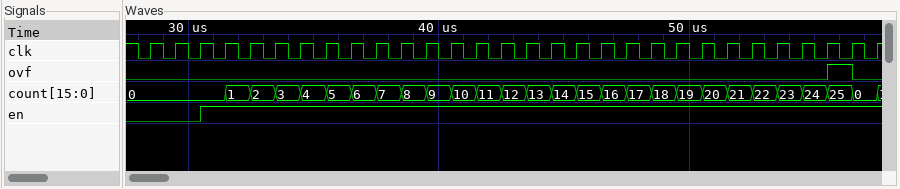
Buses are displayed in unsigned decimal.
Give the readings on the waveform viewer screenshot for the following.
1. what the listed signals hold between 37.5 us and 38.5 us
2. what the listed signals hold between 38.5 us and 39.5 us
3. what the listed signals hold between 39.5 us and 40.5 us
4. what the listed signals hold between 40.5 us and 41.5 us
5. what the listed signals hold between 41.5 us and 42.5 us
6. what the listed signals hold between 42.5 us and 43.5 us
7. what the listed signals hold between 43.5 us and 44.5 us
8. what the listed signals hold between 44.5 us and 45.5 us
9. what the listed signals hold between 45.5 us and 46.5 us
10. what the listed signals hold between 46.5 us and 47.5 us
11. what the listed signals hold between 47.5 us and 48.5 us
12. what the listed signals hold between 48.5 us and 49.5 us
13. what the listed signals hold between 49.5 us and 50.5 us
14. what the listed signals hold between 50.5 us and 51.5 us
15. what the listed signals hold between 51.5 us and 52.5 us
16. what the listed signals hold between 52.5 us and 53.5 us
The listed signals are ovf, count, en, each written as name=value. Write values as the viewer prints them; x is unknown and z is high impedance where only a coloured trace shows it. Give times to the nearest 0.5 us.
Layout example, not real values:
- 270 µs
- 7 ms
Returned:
- ovf=0, count=7, en=1
- ovf=0, count=8, en=1
- ovf=0, count=9, en=1
- ovf=0, count=10, en=1
- ovf=0, count=11, en=1
- ovf=0, count=12, en=1
- ovf=0, count=13, en=1
- ovf=0, count=14, en=1
- ovf=0, count=15, en=1
- ovf=0, count=16, en=1
- ovf=0, count=17, en=1
- ovf=0, count=18, en=1
- ovf=0, count=19, en=1
- ovf=0, count=20, en=1
- ovf=0, count=21, en=1
- ovf=0, count=22, en=1
